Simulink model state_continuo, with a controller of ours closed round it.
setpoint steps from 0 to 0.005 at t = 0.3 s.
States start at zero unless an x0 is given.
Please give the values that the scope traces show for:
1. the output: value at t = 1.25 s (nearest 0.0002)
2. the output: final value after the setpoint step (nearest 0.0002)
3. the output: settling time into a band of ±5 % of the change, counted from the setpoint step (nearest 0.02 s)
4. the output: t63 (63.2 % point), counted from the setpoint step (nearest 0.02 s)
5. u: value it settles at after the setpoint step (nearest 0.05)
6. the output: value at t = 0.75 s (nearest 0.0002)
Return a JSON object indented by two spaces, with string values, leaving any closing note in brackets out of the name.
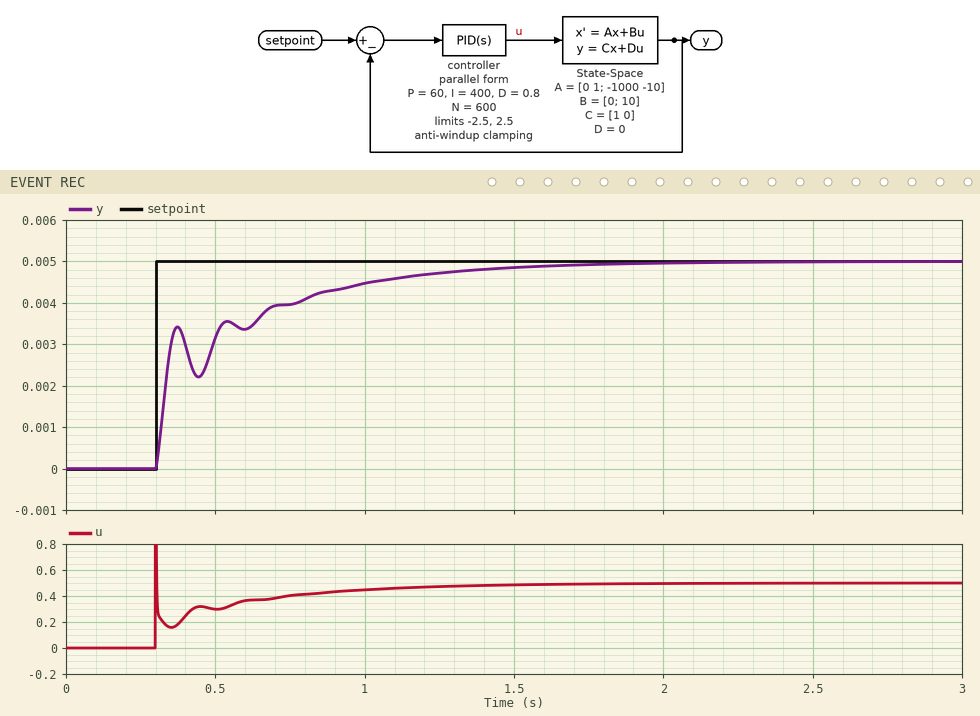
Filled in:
{
  "the output: value at t = 1.25 s": "0.0048",
  "the output: final value after the setpoint step": "0.0050",
  "the output: settling time into a band of ±5 % of the change, counted from the setpoint step": "1.00 s",
  "the output: t63 (63.2 % point), counted from the setpoint step": "0.06 s",
  "u: value it settles at after the setpoint step": "0.50",
  "the output: value at t = 0.75 s": "0.0040"
}
